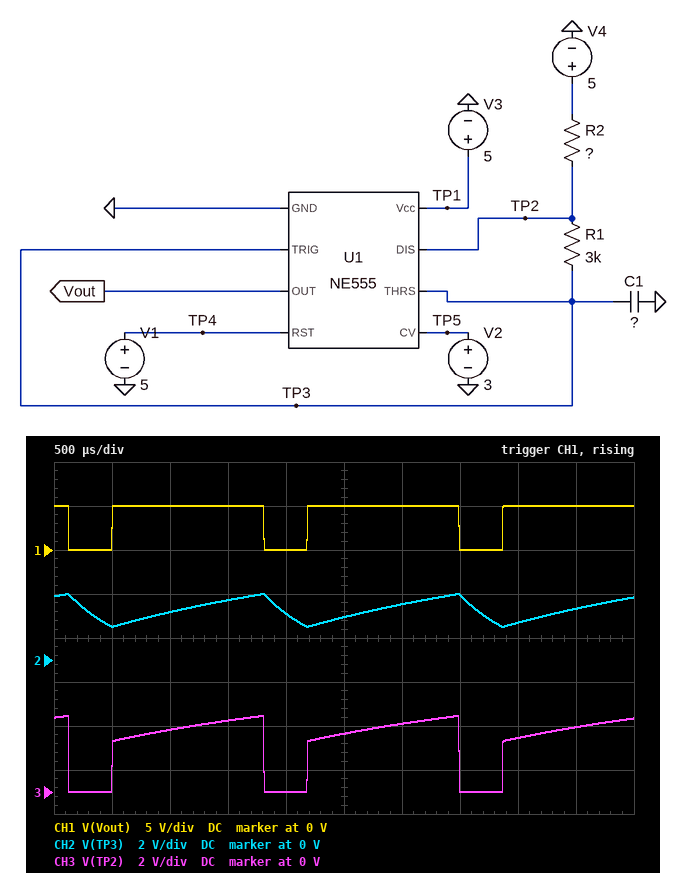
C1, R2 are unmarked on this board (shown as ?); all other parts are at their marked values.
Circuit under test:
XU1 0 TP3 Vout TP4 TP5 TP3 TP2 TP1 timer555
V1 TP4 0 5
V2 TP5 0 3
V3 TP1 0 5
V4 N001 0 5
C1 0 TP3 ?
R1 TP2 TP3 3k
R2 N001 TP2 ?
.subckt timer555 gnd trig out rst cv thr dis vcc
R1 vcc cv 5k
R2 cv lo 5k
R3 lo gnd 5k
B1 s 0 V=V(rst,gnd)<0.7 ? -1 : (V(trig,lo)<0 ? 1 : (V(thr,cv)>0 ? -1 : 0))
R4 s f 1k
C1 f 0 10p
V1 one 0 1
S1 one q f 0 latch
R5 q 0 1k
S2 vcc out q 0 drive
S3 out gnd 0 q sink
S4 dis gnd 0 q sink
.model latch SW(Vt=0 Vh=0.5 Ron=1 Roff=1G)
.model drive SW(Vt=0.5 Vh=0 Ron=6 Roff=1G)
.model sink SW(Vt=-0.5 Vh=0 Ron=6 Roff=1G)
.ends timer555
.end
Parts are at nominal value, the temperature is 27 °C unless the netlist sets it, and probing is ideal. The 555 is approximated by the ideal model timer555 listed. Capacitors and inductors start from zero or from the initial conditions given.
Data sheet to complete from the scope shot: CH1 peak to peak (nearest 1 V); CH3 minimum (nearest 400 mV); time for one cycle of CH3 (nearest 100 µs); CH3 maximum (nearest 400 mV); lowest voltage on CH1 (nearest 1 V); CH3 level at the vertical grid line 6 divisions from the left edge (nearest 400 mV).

5 V
0 V
1.7 ms
3.6 V
0 V
3.2 V
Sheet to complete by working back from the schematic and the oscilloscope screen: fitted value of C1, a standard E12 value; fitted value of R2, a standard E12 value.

180 nF
10 kΩ
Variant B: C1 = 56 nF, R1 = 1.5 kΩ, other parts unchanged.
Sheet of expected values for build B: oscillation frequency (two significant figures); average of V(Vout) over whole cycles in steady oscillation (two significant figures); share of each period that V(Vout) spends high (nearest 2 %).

2.4 kHz
4.3 V
86 %
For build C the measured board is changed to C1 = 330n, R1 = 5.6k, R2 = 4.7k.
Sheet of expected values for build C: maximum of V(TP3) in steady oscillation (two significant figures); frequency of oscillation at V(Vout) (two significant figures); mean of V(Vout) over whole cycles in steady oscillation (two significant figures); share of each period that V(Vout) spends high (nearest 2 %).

3.0 V
310 Hz
3.0 V
60 %
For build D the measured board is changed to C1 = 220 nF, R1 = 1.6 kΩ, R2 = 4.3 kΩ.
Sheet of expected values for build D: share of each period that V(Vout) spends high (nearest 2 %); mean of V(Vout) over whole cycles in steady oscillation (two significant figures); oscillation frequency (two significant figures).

74 %
3.7 V
1.0 kHz
